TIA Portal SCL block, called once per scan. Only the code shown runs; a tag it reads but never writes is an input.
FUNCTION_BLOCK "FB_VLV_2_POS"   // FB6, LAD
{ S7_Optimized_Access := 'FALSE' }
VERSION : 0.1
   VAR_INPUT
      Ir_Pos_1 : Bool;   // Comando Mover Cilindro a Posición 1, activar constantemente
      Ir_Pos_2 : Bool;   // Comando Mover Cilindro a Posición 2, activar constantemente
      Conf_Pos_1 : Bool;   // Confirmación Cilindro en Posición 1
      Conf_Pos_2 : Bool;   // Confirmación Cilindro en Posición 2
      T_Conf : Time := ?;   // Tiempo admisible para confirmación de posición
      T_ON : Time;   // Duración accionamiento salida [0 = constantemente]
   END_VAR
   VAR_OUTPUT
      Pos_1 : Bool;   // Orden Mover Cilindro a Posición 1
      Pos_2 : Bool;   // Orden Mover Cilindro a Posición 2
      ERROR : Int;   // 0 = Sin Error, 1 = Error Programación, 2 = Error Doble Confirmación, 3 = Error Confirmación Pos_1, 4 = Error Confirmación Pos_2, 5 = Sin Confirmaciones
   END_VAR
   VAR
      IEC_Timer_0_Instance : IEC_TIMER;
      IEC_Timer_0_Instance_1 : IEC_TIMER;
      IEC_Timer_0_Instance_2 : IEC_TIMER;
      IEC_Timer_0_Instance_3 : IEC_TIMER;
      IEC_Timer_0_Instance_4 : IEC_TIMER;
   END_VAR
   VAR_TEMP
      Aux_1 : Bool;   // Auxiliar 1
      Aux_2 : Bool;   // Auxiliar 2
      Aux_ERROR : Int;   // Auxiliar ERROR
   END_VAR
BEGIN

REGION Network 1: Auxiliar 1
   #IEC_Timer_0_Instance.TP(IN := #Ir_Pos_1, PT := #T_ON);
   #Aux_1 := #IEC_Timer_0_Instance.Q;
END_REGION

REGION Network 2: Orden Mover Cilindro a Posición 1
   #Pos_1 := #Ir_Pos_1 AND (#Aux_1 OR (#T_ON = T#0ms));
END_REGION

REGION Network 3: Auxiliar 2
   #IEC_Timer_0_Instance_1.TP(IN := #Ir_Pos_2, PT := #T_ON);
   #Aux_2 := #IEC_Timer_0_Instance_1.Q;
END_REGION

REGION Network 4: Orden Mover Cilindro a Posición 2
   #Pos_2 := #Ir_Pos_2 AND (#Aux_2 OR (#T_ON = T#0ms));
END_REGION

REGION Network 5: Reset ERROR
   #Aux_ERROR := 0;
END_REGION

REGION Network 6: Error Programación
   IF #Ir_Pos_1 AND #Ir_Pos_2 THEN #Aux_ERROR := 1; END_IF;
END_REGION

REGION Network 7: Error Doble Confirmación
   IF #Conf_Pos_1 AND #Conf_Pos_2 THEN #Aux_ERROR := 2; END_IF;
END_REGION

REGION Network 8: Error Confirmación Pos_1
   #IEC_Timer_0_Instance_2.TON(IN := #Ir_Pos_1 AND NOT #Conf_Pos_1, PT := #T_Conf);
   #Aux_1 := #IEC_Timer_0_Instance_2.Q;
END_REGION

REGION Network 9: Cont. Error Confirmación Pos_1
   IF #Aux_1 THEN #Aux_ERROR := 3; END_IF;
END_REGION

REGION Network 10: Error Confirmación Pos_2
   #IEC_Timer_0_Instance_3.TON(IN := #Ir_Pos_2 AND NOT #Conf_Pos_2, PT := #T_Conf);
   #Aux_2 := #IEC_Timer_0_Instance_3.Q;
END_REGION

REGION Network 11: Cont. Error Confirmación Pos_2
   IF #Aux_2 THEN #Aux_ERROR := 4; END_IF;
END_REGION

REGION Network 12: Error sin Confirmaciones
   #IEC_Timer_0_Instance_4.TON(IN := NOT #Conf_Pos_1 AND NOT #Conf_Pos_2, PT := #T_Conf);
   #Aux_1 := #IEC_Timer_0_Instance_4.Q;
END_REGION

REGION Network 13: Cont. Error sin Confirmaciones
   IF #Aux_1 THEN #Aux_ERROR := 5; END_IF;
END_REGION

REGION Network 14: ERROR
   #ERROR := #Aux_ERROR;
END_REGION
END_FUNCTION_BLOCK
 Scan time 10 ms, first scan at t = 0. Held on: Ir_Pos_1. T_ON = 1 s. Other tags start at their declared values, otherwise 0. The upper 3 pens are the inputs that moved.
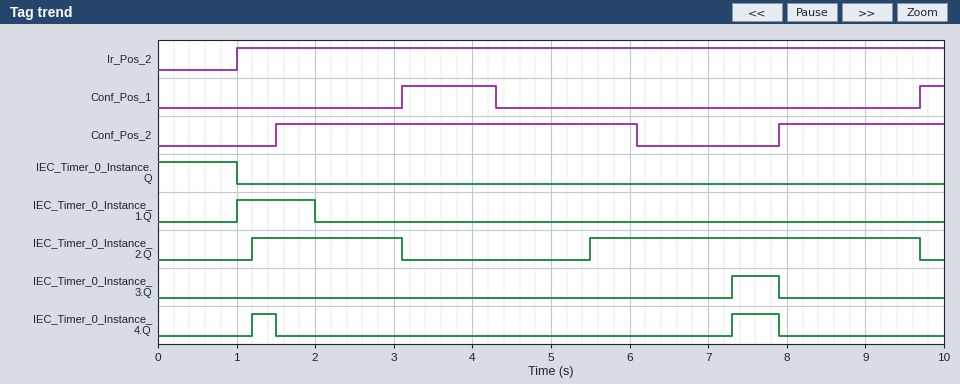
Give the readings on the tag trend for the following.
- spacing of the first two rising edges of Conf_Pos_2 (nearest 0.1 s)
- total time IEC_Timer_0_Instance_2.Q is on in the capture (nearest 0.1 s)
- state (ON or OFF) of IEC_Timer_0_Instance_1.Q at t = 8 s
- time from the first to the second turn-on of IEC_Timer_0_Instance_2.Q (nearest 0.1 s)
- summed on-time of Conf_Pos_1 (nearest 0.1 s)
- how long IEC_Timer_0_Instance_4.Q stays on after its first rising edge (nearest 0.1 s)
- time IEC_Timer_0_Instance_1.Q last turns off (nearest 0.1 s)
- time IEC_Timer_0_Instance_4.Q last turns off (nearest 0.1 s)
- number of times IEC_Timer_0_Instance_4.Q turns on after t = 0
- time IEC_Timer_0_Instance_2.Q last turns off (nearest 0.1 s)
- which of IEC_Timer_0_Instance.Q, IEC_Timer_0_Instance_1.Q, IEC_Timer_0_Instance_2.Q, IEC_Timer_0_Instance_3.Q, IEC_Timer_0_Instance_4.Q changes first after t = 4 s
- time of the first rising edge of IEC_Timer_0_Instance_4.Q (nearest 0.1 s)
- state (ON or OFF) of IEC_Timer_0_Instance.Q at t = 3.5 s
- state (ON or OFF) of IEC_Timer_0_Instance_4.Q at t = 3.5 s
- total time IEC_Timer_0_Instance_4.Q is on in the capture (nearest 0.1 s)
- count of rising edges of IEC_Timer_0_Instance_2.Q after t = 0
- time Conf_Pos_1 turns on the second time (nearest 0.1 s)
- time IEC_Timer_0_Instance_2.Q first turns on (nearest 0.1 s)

6.4 s
6.1 s
OFF
4.3 s
1.5 s
0.3 s
2.0 s
7.9 s
2
9.7 s
IEC_Timer_0_Instance_2.Q
1.2 s
OFF
OFF
0.9 s
2
9.7 s
1.2 s
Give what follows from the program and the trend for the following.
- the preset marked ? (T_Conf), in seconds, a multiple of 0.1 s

1.2 s
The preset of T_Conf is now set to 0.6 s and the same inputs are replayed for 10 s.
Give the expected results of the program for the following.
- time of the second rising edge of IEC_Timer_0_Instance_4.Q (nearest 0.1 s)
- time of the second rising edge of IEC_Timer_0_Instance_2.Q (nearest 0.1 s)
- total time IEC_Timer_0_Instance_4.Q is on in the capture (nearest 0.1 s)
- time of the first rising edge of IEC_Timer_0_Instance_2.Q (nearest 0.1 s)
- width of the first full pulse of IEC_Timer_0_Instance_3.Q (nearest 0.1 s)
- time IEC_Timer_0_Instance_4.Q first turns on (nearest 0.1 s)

6.7 s
4.9 s
2.1 s
0.6 s
1.2 s
0.6 s
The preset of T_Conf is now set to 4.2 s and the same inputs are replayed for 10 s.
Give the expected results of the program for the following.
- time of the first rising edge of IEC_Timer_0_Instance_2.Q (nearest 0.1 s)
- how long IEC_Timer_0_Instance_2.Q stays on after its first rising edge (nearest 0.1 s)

8.5 s
1.2 s
